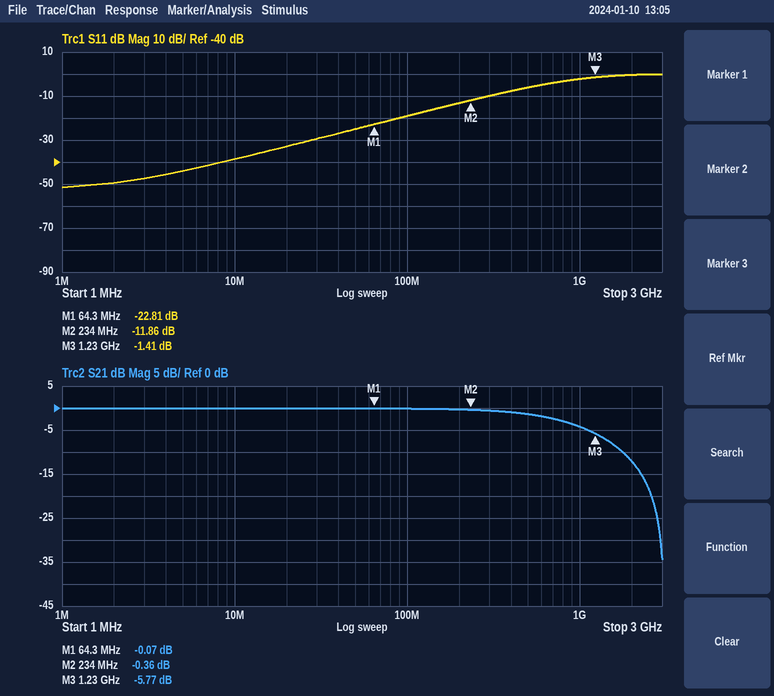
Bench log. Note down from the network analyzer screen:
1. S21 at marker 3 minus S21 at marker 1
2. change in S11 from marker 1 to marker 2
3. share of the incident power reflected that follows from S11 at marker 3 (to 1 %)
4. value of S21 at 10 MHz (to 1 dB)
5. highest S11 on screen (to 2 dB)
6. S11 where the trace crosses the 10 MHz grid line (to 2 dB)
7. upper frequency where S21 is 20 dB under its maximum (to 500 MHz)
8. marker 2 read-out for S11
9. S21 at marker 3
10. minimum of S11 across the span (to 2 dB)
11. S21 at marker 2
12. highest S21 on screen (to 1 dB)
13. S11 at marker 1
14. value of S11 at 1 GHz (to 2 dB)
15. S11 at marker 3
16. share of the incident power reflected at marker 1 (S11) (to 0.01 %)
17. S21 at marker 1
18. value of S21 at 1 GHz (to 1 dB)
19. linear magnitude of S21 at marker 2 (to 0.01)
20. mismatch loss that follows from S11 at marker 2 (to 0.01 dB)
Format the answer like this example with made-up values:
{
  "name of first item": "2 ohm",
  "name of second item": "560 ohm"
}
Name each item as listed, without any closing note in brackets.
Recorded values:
{
  "S21 at marker 3 minus S21 at marker 1": "-5.70 dB",
  "change in S11 from marker 1 to marker 2": "10.95 dB",
  "share of the incident power reflected that follows from S11 at marker 3": "72 %",
  "value of S21 at 10 MHz": "0 dB",
  "highest S11 on screen": "0 dB",
  "S11 where the trace crosses the 10 MHz grid line": "-38 dB",
  "upper frequency where S21 is 20 dB under its maximum": "2.5 GHz",
  "marker 2 read-out for S11": "-11.86 dB",
  "S21 at marker 3": "-5.77 dB",
  "minimum of S11 across the span": "-52 dB",
  "S21 at marker 2": "-0.36 dB",
  "highest S21 on screen": "0 dB",
  "S11 at marker 1": "-22.81 dB",
  "value of S11 at 1 GHz": "-2 dB",
  "S11 at marker 3": "-1.41 dB",
  "share of the incident power reflected at marker 1 (S11)": "0.52 %",
  "S21 at marker 1": "-0.07 dB",
  "value of S21 at 1 GHz": "-4 dB",
  "linear magnitude of S21 at marker 2": "0.96",
  "mismatch loss that follows from S11 at marker 2": "0.29 dB"
}
